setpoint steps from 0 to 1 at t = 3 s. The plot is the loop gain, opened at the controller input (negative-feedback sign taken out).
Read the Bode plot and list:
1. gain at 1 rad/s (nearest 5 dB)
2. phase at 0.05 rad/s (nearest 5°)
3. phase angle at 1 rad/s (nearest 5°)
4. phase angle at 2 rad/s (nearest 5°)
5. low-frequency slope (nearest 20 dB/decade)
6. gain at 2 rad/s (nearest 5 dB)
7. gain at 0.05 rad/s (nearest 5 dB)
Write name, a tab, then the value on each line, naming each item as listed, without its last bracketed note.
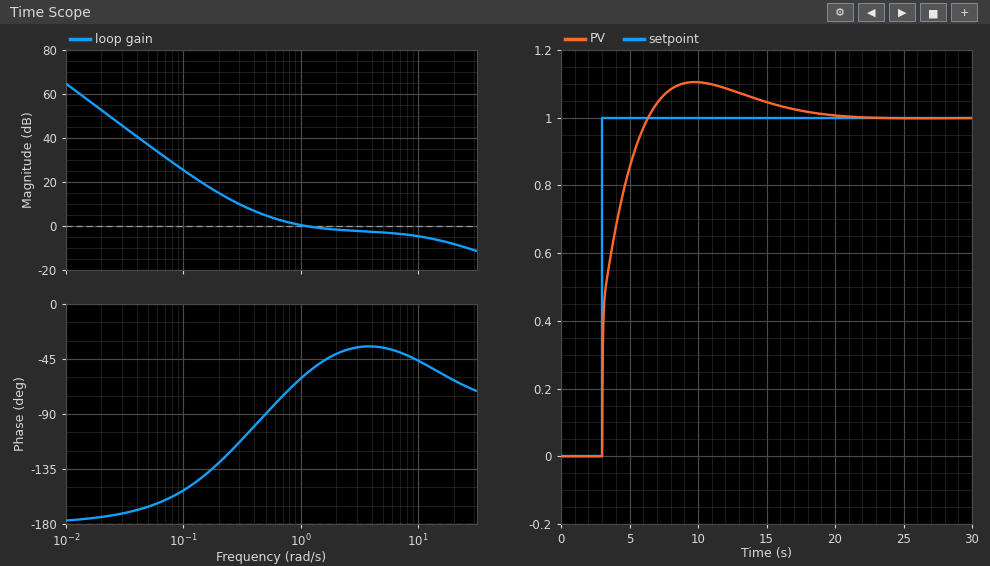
gain at 1 rad/s	0 dB
phase at 0.05 rad/s	-165°
phase angle at 1 rad/s	-60°
phase angle at 2 rad/s	-40°
low-frequency slope	-40 dB/decade
gain at 2 rad/s	0 dB
gain at 0.05 rad/s	35 dB
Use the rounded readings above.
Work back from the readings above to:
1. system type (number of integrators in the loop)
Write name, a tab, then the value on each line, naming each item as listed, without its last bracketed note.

system type	2
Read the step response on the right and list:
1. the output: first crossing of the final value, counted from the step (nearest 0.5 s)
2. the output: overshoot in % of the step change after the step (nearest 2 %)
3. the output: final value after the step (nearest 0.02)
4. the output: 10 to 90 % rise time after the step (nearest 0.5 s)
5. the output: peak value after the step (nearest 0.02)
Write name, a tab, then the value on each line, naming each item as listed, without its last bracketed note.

the output: first crossing of the final value, counted from the step	3.5 s
the output: overshoot in % of the step change after the step	10 %
the output: final value after the step	1.00
the output: 10 to 90 % rise time after the step	2.5 s
the output: peak value after the step	1.10
